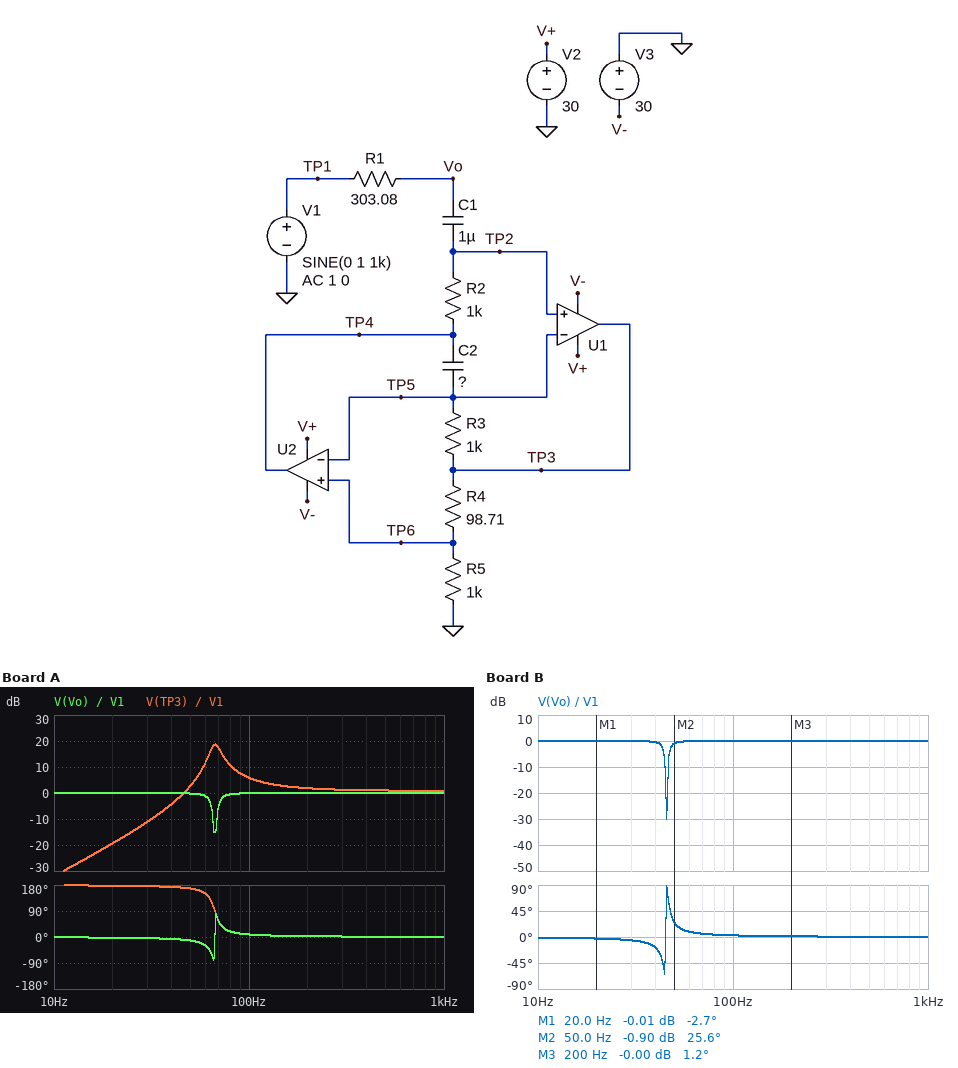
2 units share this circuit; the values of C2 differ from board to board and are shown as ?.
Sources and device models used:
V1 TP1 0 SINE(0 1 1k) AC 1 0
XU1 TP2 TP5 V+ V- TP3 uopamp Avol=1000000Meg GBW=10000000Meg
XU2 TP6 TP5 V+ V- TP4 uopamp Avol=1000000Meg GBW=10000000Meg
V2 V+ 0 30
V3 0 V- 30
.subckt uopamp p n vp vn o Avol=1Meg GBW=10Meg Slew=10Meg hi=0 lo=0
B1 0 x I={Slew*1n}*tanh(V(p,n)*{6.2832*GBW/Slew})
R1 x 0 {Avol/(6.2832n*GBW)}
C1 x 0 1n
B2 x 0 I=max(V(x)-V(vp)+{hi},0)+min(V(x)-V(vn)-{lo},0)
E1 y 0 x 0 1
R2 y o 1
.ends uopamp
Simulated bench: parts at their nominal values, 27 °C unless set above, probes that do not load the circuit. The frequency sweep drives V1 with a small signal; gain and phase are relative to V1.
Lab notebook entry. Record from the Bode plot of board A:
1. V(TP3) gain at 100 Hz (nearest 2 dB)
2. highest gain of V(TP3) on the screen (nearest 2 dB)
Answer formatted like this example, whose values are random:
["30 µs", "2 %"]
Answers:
["6 dB", "18 dB"]
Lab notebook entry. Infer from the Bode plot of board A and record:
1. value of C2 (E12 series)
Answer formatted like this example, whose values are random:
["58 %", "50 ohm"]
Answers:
["560 nF"]
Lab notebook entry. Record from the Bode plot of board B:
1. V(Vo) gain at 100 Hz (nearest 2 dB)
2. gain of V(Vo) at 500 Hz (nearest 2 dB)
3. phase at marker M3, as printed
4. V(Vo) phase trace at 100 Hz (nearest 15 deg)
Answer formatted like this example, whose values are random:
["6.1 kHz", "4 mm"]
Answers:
["0 dB", "0 dB", "1.2 deg", "0 deg"]
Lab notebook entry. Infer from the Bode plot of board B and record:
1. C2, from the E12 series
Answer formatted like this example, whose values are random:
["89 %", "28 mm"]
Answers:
["1.2 µF"]
